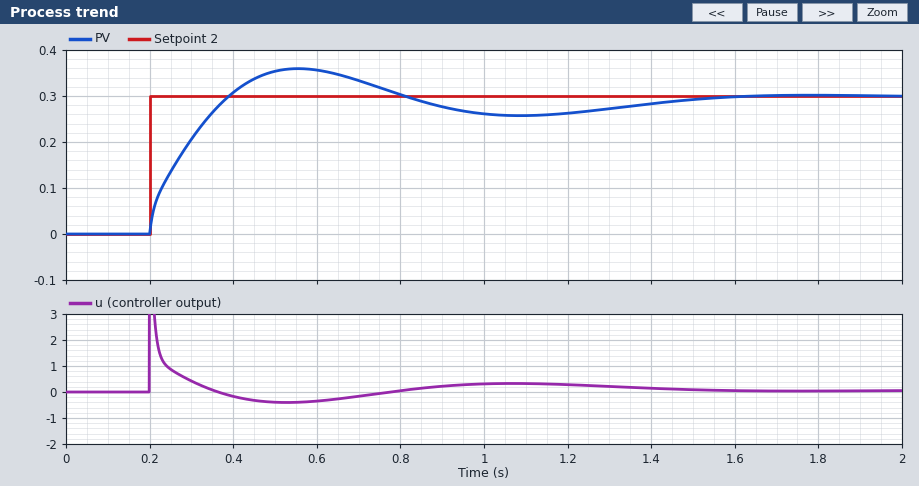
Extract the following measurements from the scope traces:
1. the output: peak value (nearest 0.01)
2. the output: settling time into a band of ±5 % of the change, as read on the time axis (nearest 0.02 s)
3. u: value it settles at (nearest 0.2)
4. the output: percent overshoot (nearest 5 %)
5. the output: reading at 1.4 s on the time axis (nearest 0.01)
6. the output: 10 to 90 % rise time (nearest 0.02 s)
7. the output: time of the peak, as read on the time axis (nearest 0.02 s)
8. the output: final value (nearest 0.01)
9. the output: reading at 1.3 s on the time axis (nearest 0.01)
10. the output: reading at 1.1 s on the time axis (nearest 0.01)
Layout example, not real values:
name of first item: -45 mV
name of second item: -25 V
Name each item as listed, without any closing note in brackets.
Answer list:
the output: peak value: 0.36
the output: settling time into a band of ±5 % of the change, as read on the time axis: 1.42 s
u: value it settles at: 0.0
the output: percent overshoot: 20 %
the output: reading at 1.4 s on the time axis: 0.28
the output: 10 to 90 % rise time: 0.16 s
the output: time of the peak, as read on the time axis: 0.56 s
the output: final value: 0.30
the output: reading at 1.3 s on the time axis: 0.27
the output: reading at 1.1 s on the time axis: 0.26
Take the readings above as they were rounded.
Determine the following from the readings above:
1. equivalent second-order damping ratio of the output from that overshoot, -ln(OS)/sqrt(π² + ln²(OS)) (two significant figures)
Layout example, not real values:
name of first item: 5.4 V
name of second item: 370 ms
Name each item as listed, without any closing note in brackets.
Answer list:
equivalent second-order damping ratio of the output from that overshoot, -ln(OS)/sqrt(π² + ln²(OS)): 0.46
